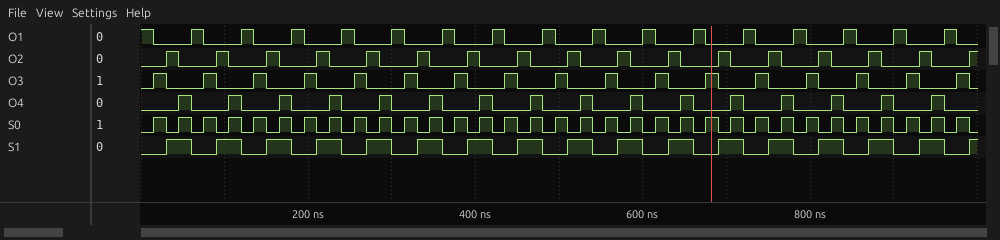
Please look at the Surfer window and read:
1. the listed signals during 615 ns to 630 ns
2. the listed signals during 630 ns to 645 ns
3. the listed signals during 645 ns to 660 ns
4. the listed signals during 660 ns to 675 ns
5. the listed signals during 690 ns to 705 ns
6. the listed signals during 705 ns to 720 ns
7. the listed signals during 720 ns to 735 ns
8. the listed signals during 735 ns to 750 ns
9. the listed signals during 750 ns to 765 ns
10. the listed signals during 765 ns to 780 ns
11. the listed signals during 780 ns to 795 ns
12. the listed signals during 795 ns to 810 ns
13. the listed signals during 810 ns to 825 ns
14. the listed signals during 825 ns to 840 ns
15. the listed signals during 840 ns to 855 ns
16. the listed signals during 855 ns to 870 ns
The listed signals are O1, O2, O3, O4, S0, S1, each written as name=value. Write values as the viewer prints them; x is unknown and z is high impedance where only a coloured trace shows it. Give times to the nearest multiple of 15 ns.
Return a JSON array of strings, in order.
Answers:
["O1=0, O2=0, O3=1, O4=0, S0=1, S1=0", "O1=0, O2=1, O3=0, O4=0, S0=0, S1=1", "O1=0, O2=0, O3=0, O4=1, S0=1, S1=1", "O1=1, O2=0, O3=0, O4=0, S0=0, S1=0", "O1=0, O2=1, O3=0, O4=0, S0=0, S1=1", "O1=0, O2=0, O3=0, O4=1, S0=1, S1=1", "O1=1, O2=0, O3=0, O4=0, S0=0, S1=0", "O1=0, O2=0, O3=1, O4=0, S0=1, S1=0", "O1=0, O2=1, O3=0, O4=0, S0=0, S1=1", "O1=0, O2=0, O3=0, O4=1, S0=1, S1=1", "O1=1, O2=0, O3=0, O4=0, S0=0, S1=0", "O1=0, O2=0, O3=1, O4=0, S0=1, S1=0", "O1=0, O2=1, O3=0, O4=0, S0=0, S1=1", "O1=0, O2=0, O3=0, O4=1, S0=1, S1=1", "O1=1, O2=0, O3=0, O4=0, S0=0, S1=0", "O1=0, O2=0, O3=1, O4=0, S0=1, S1=0"]
